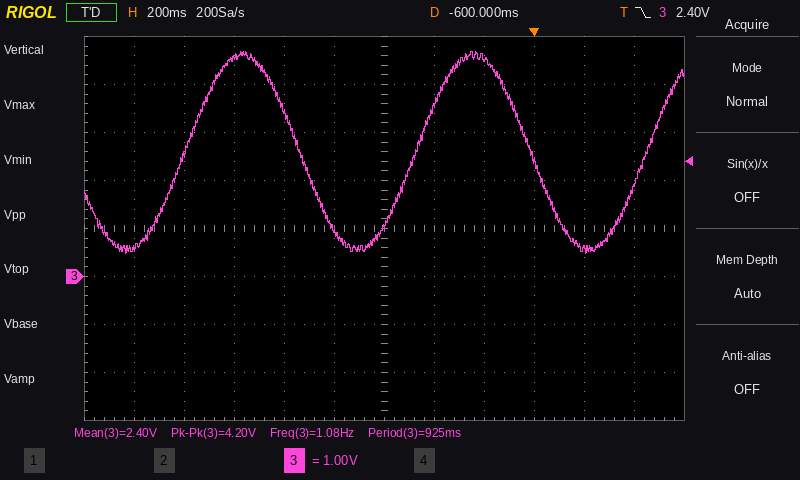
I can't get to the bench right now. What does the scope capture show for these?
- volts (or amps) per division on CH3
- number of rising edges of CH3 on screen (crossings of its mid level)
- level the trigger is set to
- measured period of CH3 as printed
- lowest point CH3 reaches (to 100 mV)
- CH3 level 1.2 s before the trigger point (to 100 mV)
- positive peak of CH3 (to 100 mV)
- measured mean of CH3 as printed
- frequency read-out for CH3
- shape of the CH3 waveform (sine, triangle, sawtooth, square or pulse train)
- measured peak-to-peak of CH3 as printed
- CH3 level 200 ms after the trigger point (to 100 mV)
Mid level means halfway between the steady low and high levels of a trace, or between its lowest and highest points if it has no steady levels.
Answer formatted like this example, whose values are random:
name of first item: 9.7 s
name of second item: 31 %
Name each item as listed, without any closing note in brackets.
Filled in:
volts (or amps) per division on CH3: 1 V
number of rising edges of CH3 on screen: 3
level the trigger is set to: 2.40 V
measured period of CH3 as printed: 925 ms
lowest point CH3 reaches: 500 mV
CH3 level 1.2 s before the trigger point: 4.6 V
positive peak of CH3: 4.7 V
measured mean of CH3 as printed: 2.40 V
frequency read-out for CH3: 1.08 Hz
shape of the CH3 waveform: sine
measured peak-to-peak of CH3 as printed: 4.20 V
CH3 level 200 ms after the trigger point: 600 mV
